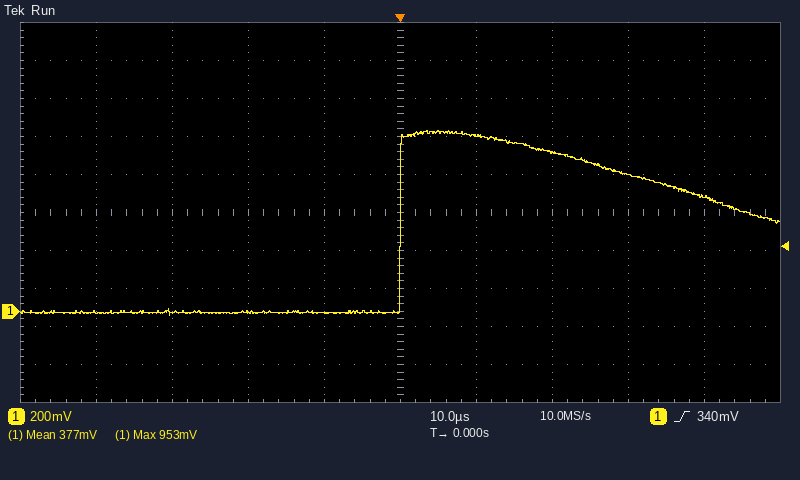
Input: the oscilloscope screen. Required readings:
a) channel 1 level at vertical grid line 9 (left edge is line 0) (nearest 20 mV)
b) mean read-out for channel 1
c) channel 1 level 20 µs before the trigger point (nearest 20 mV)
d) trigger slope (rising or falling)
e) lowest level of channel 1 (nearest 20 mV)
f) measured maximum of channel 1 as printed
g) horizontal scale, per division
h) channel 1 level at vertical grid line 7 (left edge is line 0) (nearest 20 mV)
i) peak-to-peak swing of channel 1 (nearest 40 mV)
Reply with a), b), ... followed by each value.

a) 600 mV
b) 377 mV
c) 0 mV
d) rising
e) -20 mV
f) 953 mV
g) 10 µs
h) 840 mV
i) 960 mV
